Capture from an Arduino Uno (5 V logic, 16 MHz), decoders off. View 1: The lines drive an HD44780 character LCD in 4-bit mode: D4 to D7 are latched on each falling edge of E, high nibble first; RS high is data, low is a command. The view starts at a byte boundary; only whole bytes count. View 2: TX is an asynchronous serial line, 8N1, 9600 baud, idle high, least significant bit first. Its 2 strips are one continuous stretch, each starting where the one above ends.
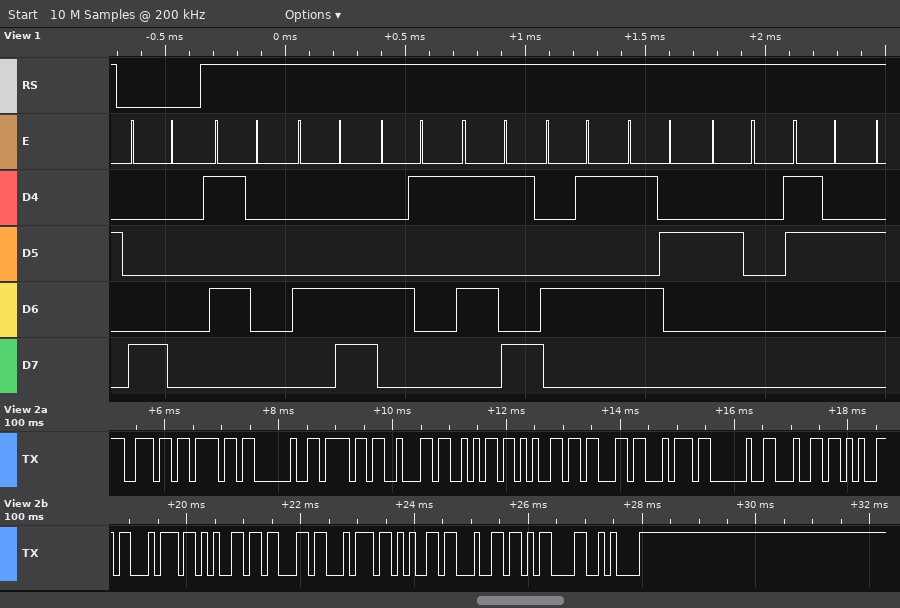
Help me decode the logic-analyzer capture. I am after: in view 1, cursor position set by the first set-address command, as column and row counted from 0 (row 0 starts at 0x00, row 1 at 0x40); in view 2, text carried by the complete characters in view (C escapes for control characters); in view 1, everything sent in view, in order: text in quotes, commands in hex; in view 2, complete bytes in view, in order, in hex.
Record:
column 0, row 0
"no object detected\r\n"
0x80 "PLAYER 2"
6E 6F 20 6F 62 6A 65 63 74 20 64 65 74 65 63 74 65 64 0D 0A
